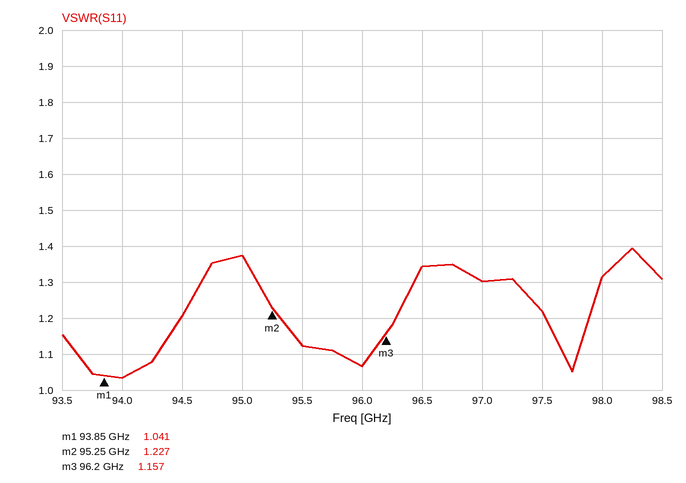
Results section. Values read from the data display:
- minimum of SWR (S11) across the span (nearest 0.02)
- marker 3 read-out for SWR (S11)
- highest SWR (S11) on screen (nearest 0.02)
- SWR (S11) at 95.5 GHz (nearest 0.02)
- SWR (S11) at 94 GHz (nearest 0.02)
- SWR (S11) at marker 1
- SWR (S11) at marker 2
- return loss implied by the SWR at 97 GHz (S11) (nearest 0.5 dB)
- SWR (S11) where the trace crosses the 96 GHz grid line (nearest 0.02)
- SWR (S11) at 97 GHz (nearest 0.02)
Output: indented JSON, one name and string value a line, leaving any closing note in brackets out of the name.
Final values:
{
  "minimum of SWR (S11) across the span": "1.04",
  "marker 3 read-out for SWR": "1.157",
  "highest SWR (S11) on screen": "1.40",
  "SWR (S11) at 95.5 GHz": "1.12",
  "SWR (S11) at 94 GHz": "1.04",
  "SWR (S11) at marker 1": "1.041",
  "SWR (S11) at marker 2": "1.227",
  "return loss implied by the SWR at 97 GHz (S11)": "17.5 dB",
  "SWR (S11) where the trace crosses the 96 GHz grid line": "1.06",
  "SWR (S11) at 97 GHz": "1.30"
}
